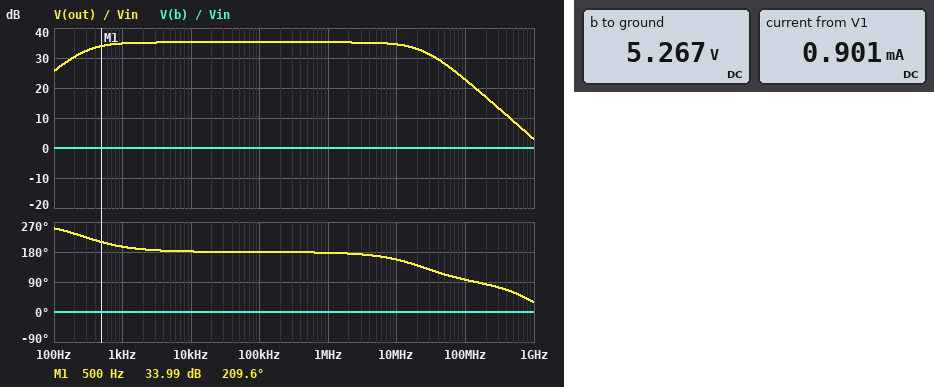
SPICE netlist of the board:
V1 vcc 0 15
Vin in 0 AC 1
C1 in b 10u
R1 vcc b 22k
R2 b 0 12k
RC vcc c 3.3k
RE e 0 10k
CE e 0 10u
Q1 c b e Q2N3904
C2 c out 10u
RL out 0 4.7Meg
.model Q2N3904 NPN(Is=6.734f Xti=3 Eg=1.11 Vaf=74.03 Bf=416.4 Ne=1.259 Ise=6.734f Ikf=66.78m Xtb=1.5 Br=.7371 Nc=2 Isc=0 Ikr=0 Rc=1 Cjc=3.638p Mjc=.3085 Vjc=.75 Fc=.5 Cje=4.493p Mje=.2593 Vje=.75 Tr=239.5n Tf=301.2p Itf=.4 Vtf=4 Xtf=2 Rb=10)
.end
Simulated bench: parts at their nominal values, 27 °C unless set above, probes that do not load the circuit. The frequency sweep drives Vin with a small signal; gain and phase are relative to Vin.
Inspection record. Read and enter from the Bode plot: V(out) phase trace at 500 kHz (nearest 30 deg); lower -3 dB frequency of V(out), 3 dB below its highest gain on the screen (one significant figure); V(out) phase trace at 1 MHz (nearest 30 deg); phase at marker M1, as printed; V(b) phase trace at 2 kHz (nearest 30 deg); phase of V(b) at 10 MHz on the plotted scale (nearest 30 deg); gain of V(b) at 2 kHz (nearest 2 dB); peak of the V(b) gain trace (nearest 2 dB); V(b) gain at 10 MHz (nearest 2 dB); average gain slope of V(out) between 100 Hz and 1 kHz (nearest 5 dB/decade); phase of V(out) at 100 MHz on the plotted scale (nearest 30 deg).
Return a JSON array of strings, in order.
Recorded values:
["180 deg", "300 Hz", "180 deg", "209.6 deg", "0 deg", "0 deg", "0 dB", "0 dB", "0 dB", "10 dB/decade", "90 deg"]
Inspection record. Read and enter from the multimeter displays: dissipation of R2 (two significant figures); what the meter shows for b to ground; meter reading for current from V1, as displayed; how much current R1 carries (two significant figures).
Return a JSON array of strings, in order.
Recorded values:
["2.3 mW", "5.267 V", "0.901 mA", "440 µA"]
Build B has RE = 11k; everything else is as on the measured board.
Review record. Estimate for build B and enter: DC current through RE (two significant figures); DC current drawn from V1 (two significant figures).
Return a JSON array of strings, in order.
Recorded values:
["420 µA", "860 µA"]
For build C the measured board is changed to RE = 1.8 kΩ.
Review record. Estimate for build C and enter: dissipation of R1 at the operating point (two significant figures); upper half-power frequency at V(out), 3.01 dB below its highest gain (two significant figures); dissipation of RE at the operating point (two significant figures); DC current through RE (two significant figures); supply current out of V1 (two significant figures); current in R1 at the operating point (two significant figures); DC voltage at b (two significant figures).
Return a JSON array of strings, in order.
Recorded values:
["4.4 mW", "11 MHz", "11 mW", "2.5 mA", "2.9 mA", "450 µA", "5.2 V"]
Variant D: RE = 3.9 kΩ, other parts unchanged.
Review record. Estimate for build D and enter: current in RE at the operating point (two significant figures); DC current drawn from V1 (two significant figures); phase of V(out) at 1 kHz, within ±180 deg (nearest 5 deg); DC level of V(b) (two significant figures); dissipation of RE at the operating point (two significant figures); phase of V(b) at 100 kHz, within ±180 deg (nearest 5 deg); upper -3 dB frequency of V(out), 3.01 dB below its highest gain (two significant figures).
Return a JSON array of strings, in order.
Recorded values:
["1.2 mA", "1.6 mA", "-145 deg", "5.2 V", "5.3 mW", "0 deg", "19 MHz"]
